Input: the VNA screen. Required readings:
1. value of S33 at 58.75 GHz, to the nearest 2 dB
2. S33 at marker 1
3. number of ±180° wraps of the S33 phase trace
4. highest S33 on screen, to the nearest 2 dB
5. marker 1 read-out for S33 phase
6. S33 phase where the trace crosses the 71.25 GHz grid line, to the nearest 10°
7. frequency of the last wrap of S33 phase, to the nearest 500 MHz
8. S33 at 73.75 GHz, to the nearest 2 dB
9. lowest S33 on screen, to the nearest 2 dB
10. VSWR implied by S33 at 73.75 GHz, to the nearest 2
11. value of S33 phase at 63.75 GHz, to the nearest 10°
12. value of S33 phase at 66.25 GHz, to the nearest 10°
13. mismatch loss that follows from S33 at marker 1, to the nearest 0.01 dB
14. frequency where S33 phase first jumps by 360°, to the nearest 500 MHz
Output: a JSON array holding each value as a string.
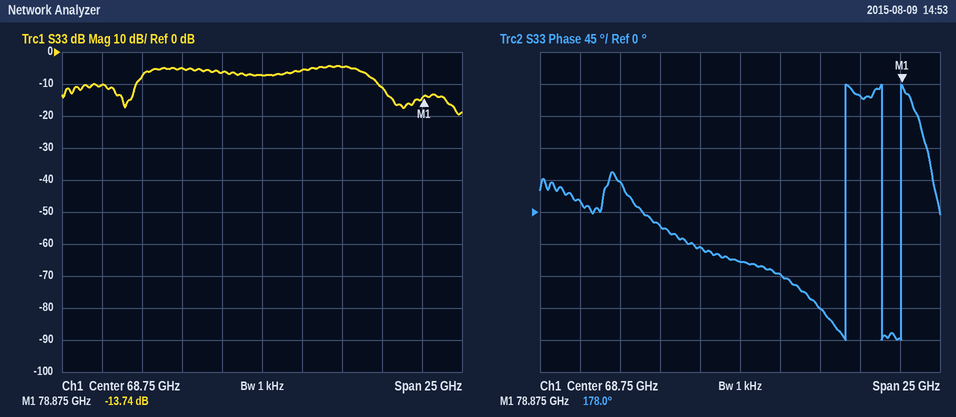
["-10 dB", "-13.74 dB", "3", "-4 dB", "178.0°", "-90°", "79.0 GHz", "-4 dB", "-20 dB", "4", "-20°", "-50°", "0.19 dB", "75.5 GHz"]
